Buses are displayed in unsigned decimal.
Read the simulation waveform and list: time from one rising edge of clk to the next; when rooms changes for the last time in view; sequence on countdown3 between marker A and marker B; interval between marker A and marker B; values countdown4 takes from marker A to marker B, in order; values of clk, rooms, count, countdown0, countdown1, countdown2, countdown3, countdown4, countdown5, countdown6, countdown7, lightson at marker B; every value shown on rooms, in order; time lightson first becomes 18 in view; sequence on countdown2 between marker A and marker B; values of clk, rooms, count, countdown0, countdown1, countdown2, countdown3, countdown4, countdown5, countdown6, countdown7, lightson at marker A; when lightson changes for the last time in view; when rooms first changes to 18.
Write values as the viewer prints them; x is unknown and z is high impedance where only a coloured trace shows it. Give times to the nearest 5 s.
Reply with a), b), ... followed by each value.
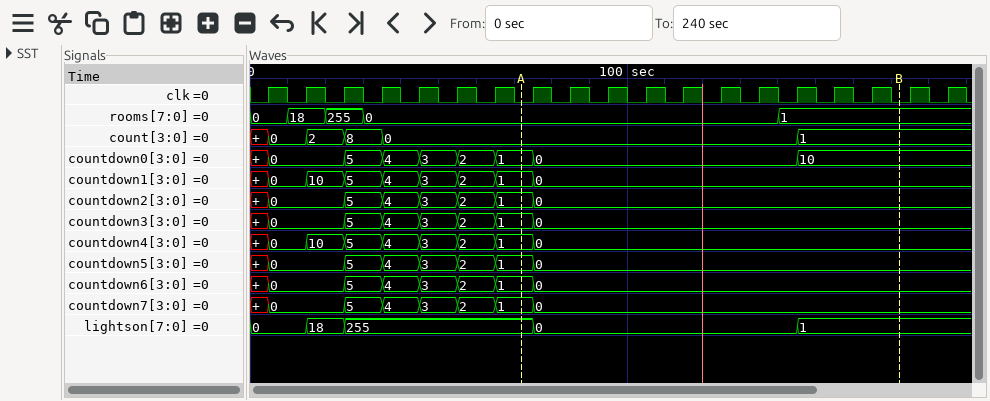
a) 10 s
b) 140 s
c) 1, 0
d) 100 s
e) 1, 0
f) clk=0, rooms=1, count=1, countdown0=10, countdown1=0, countdown2=0, countdown3=0, countdown4=0, countdown5=0, countdown6=0, countdown7=0, lightson=1
g) 0, 18, 255, 0, 1
h) 15 s
i) 1, 0
j) clk=0, rooms=0, count=0, countdown0=1, countdown1=1, countdown2=1, countdown3=1, countdown4=1, countdown5=1, countdown6=1, countdown7=1, lightson=255
k) 145 s
l) 10 s
